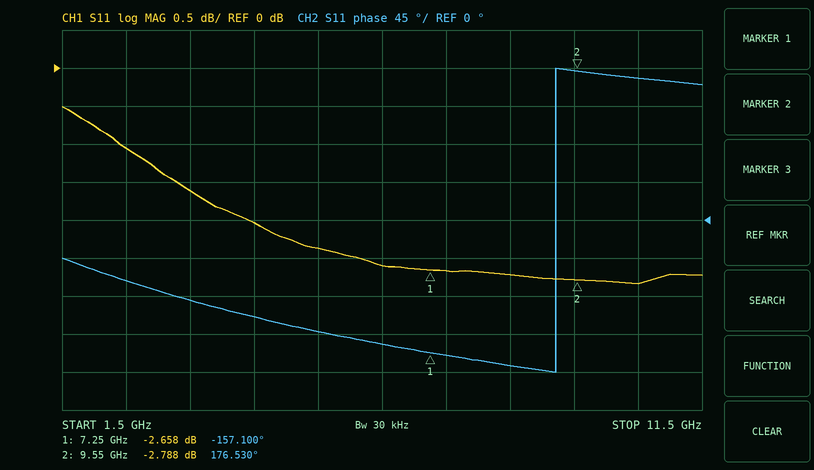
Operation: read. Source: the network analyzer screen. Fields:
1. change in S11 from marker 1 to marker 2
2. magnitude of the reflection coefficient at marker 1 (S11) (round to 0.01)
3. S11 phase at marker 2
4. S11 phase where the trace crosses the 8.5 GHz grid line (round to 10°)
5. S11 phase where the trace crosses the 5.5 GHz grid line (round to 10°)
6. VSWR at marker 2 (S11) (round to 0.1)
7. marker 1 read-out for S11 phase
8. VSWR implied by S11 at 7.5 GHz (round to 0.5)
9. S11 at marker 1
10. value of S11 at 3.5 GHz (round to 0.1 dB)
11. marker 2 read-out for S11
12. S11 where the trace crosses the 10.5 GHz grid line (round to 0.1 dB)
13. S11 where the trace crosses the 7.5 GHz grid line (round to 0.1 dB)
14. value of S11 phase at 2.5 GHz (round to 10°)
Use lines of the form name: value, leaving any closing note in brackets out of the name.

change in S11 from marker 1 to marker 2: -0.130 dB
magnitude of the reflection coefficient at marker 1 (S11): 0.74
S11 phase at marker 2: 176.530°
S11 phase where the trace crosses the 8.5 GHz grid line: -170°
S11 phase where the trace crosses the 5.5 GHz grid line: -130°
VSWR at marker 2 (S11): 6.3
marker 1 read-out for S11 phase: -157.100°
VSWR implied by S11 at 7.5 GHz: 6.5
S11 at marker 1: -2.658 dB
value of S11 at 3.5 GHz: -1.6 dB
marker 2 read-out for S11: -2.788 dB
S11 where the trace crosses the 10.5 GHz grid line: -2.8 dB
S11 where the trace crosses the 7.5 GHz grid line: -2.7 dB
value of S11 phase at 2.5 GHz: -70°
